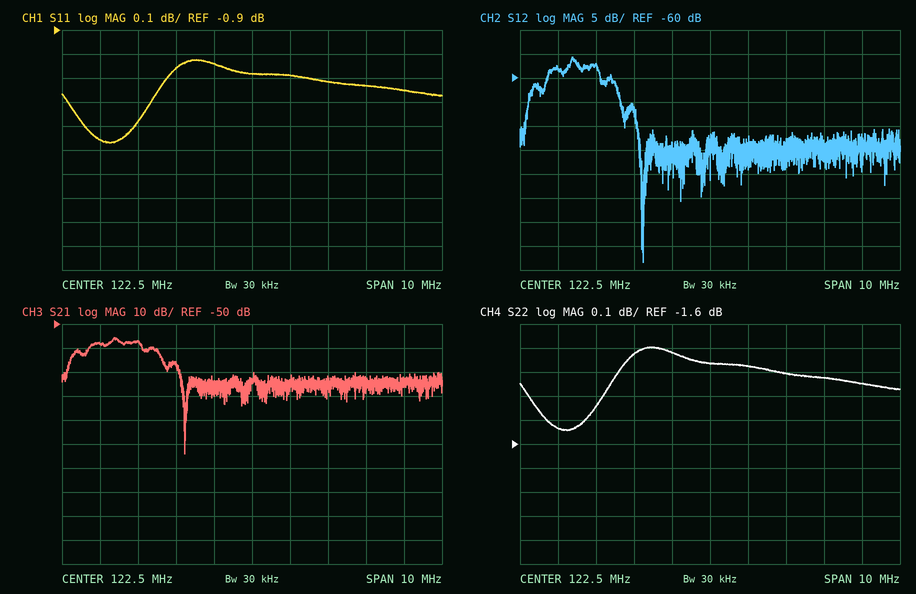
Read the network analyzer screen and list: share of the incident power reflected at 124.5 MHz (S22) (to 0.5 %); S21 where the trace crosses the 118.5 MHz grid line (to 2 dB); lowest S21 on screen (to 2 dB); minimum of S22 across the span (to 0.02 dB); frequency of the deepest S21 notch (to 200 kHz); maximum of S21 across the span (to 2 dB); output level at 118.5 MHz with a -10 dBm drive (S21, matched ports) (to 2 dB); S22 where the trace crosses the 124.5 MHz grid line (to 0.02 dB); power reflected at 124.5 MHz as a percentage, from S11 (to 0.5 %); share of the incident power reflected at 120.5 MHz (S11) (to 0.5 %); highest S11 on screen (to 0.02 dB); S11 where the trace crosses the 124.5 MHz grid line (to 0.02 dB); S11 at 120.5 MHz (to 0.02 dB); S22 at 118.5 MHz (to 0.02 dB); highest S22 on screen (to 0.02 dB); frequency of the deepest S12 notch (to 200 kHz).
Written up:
74.0 %
-58 dB
-104 dB
-1.54 dB
120.8 MHz
-56 dB
-68 dBm
-1.30 dB
77.5 %
78.5 %
-1.02 dB
-1.12 dB
-1.06 dB
-1.54 dB
-1.20 dB
120.8 MHz
